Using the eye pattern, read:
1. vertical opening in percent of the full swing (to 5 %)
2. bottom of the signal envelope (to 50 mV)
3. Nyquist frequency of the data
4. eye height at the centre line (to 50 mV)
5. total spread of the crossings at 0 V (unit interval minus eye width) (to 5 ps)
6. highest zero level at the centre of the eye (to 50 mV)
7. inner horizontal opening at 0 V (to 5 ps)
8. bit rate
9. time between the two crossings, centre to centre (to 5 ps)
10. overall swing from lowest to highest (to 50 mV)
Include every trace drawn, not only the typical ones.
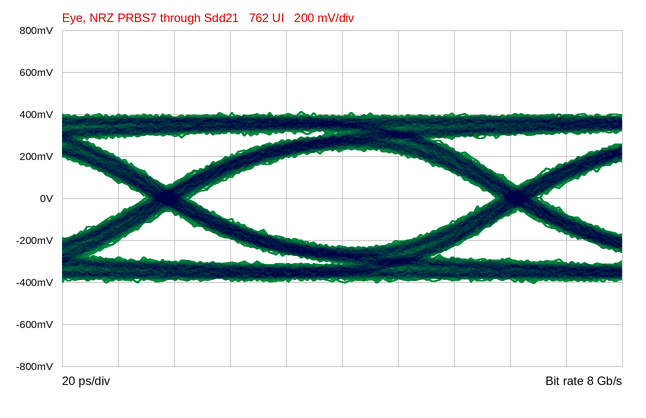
55 %
-400 mV
4 GHz
450 mV
15 ps
-250 mV
110 ps
8 Gb/s
125 ps
800 mV
